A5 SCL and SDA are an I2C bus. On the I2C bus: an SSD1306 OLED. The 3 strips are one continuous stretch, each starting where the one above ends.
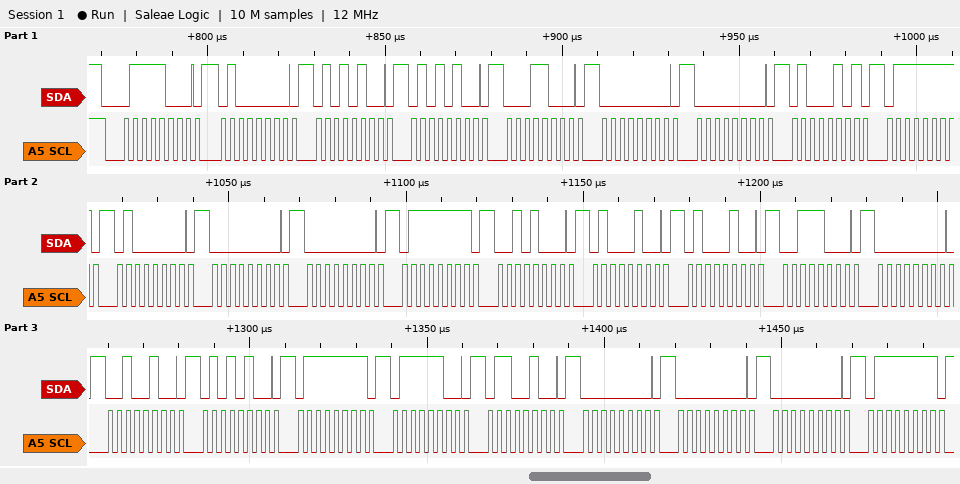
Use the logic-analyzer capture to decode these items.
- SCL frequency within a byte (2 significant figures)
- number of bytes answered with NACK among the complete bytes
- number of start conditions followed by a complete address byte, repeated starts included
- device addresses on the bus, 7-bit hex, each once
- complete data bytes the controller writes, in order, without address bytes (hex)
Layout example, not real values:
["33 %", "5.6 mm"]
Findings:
["400 kHz", "0", "1", "0x3C", "40 54 54 18 00 00 45 7F 40 00 00 7F 28 44 44 38 00 24 54 7F 7C 64 00 00 00 7F"]
